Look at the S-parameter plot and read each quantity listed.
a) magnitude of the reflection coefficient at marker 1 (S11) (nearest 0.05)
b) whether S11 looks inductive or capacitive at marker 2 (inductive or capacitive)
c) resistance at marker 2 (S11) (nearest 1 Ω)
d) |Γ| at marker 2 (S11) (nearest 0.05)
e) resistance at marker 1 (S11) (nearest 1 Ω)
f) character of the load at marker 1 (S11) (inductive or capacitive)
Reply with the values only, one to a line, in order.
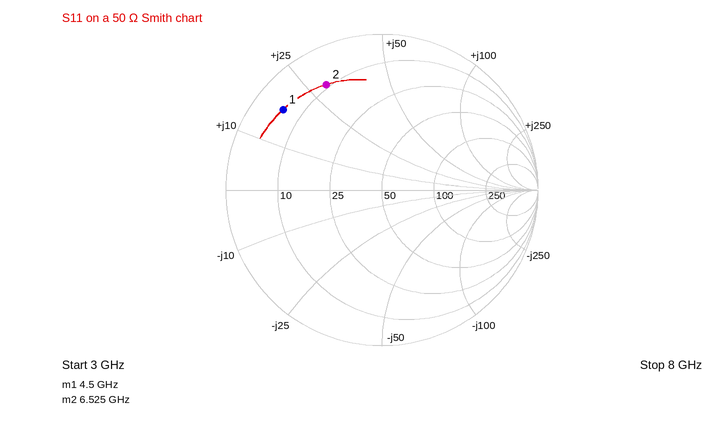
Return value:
0.80
inductive
9 Ω
0.75
6 Ω
inductive
